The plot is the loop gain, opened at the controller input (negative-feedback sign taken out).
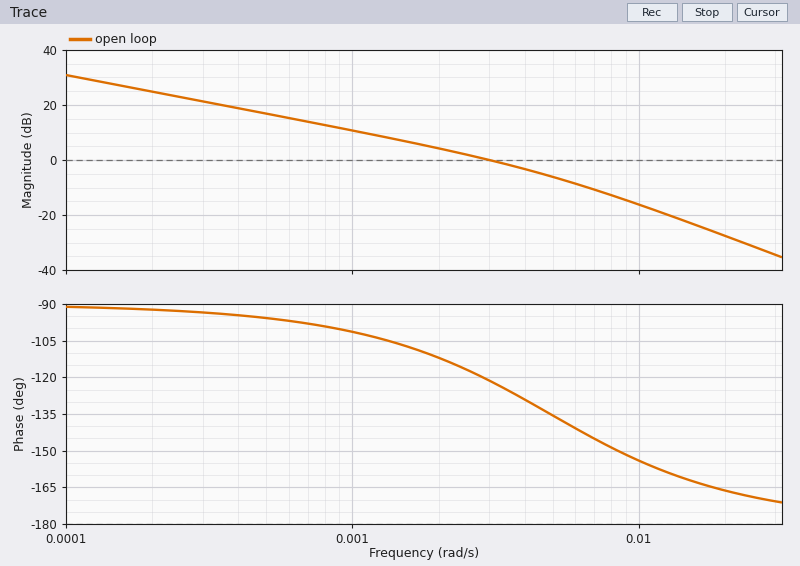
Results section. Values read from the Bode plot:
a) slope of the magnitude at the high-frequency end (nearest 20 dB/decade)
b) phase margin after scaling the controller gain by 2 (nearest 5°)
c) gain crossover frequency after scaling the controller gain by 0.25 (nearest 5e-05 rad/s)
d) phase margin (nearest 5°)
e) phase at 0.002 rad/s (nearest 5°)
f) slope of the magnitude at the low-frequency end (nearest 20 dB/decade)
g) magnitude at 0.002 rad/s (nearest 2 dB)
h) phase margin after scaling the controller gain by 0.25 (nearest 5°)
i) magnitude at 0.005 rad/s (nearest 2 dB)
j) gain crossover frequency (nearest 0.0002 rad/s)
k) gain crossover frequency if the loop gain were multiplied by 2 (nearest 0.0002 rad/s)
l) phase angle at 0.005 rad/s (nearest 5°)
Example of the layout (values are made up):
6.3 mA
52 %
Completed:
-40 dB/decade
45°
0.00085 rad/s
60°
-110°
-20 dB/decade
4 dB
80°
-6 dB
0.0030 rad/s
0.0050 rad/s
-135°
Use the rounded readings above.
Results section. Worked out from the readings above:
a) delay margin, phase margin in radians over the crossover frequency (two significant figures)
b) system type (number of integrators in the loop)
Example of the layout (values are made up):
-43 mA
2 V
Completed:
350 s
1
